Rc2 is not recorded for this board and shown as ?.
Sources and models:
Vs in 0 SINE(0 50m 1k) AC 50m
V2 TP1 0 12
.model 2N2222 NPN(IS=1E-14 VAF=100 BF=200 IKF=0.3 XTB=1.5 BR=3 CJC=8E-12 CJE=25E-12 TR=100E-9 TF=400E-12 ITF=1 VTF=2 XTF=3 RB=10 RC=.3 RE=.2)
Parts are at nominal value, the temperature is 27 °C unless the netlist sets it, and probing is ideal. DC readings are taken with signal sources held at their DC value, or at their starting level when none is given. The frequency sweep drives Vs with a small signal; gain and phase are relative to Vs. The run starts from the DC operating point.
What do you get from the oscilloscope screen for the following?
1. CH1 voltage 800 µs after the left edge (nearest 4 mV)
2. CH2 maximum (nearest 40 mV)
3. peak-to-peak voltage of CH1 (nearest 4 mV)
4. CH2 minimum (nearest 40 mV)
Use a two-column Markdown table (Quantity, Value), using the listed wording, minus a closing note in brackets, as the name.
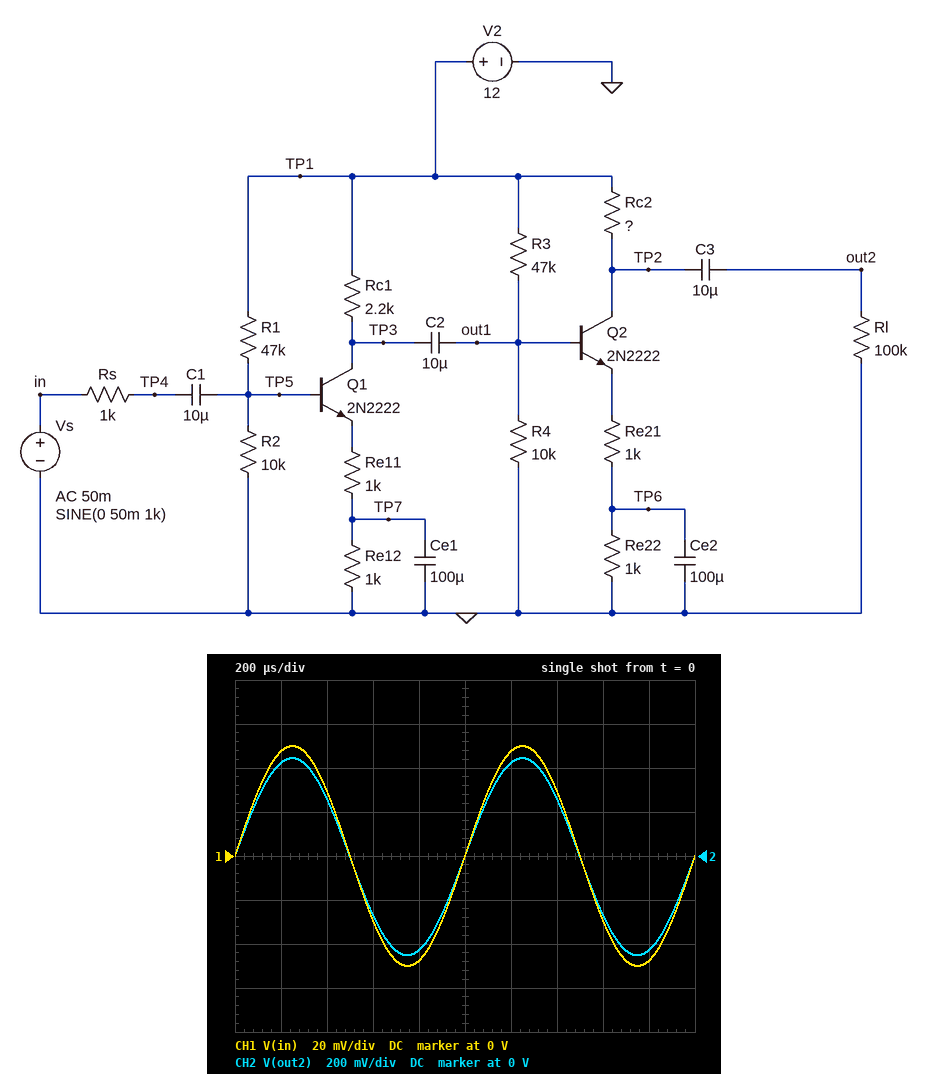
| Quantity | Value |
|---|---|
| CH1 voltage 800 µs after the left edge | -48 mV |
| CH2 maximum | 440 mV |
| peak-to-peak voltage of CH1 | 100 mV |
| CH2 minimum | -440 mV |
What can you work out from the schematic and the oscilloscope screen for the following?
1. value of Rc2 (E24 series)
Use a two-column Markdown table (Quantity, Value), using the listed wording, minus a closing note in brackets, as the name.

| Quantity | Value |
|---|---|
| value of Rc2 | 6.8 kΩ |
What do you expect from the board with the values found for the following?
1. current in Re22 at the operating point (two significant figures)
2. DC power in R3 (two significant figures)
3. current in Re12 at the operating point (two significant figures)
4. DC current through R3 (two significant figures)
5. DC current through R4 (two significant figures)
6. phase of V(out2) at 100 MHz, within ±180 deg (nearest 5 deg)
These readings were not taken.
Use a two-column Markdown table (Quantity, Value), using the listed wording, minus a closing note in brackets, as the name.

| Quantity | Value |
|---|---|
| current in Re22 at the operating point | 720 µA |
| DC power in R3 | 2.1 mW |
| current in Re12 at the operating point | 720 µA |
| DC current through R3 | 210 µA |
| DC current through R4 | 210 µA |
| phase of V(out2) at 100 MHz, within ±180 deg | 35 deg |
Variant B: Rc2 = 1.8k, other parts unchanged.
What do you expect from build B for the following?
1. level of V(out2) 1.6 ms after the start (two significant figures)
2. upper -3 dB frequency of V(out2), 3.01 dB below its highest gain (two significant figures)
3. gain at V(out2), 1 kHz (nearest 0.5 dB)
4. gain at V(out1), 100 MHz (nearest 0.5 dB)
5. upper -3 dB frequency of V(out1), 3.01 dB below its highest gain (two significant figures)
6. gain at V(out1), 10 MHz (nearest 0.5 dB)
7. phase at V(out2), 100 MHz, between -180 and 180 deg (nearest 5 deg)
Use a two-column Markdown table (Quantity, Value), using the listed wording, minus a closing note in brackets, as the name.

| Quantity | Value |
|---|---|
| level of V(out2) 1.6 ms after the start | -75 mV |
| upper -3 dB frequency of V(out2), 3.01 dB below its highest gain | 4.4 MHz |
| gain at V(out2), 1 kHz | 8.0 dB |
| gain at V(out1), 100 MHz | -12.5 dB |
| upper -3 dB frequency of V(out1), 3.01 dB below its highest gain | 4.5 MHz |
| gain at V(out1), 10 MHz | -4.0 dB |
| phase at V(out2), 100 MHz, between -180 and 180 deg | 45 deg |
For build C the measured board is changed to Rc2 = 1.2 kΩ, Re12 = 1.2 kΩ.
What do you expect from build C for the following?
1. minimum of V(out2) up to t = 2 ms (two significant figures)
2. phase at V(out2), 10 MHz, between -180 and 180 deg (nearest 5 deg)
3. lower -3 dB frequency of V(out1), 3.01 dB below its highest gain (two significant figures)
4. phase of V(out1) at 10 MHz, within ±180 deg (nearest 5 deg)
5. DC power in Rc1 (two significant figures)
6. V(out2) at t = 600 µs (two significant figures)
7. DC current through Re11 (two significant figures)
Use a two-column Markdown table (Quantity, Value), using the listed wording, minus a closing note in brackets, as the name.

| Quantity | Value |
|---|---|
| minimum of V(out2) up to t = 2 ms | -84 mV |
| phase at V(out2), 10 MHz, between -180 and 180 deg | -115 deg |
| lower -3 dB frequency of V(out1), 3.01 dB below its highest gain | 3.8 Hz |
| phase of V(out1) at 10 MHz, within ±180 deg | 95 deg |
| DC power in Rc1 | 930 µW |
| V(out2) at t = 600 µs | -50 mV |
| DC current through Re11 | 650 µA |
